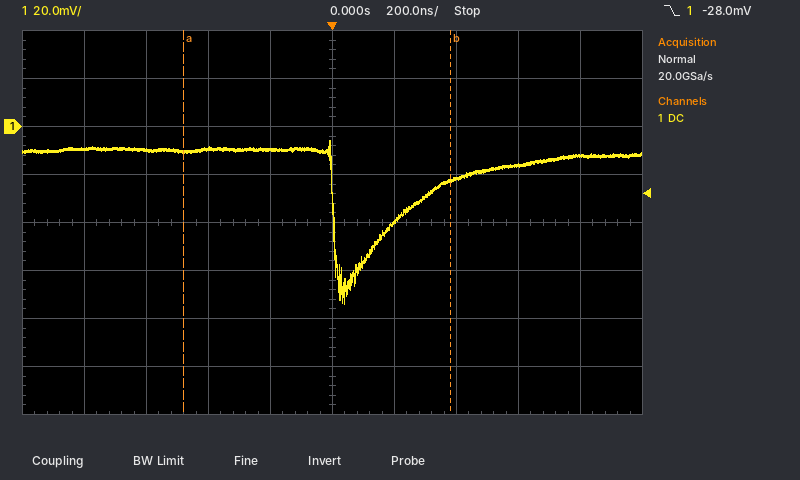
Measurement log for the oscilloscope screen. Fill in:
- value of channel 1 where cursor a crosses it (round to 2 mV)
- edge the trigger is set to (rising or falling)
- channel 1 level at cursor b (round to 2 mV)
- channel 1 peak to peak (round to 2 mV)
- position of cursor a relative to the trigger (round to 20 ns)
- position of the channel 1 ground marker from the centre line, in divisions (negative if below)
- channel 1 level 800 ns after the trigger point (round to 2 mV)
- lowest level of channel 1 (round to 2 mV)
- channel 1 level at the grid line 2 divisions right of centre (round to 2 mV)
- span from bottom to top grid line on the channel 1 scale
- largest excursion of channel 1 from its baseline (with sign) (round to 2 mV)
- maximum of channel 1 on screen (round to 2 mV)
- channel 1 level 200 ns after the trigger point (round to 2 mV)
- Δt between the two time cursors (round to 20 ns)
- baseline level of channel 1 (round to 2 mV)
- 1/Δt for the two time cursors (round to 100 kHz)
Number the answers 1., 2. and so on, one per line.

1. -10 mV
2. falling
3. -22 mV
4. 68 mV
5. -480 ns
6. +2.0 div
7. -12 mV
8. -74 mV
9. -22 mV
10. 160 mV
11. -64 mV
12. -6 mV
13. -40 mV
14. 860 ns
15. -10 mV
16. 1.2 MHz
